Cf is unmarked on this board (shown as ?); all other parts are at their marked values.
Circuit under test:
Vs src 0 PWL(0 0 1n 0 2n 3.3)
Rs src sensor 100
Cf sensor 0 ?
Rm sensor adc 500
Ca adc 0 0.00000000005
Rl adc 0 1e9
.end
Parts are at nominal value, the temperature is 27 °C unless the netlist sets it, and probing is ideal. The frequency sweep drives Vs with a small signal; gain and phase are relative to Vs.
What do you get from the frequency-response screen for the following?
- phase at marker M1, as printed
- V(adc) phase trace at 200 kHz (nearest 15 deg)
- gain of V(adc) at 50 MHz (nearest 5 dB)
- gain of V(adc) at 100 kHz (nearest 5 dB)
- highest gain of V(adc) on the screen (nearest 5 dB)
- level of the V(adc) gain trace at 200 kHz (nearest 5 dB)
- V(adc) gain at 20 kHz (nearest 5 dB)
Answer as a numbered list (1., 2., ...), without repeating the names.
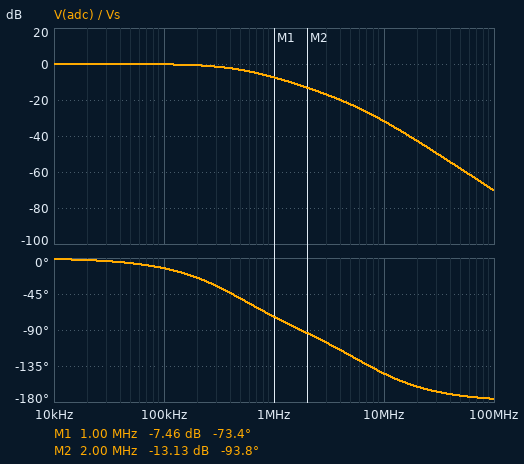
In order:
1. -73.4 deg
2. -30 deg
3. -60 dB
4. 0 dB
5. 0 dB
6. 0 dB
7. 0 dB
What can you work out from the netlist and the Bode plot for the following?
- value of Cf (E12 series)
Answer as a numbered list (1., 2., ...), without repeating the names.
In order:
1. 3.3 nF
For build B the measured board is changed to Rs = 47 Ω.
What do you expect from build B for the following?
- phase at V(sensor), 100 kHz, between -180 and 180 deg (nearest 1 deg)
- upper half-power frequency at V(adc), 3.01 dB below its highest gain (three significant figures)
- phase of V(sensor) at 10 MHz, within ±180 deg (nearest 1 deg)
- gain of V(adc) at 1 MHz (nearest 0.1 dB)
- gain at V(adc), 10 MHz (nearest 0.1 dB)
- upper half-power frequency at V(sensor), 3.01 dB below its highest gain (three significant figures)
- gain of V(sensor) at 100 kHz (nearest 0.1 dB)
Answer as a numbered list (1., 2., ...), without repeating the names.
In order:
1. -6 deg
2. 985 kHz
3. -84 deg
4. -3.1 dB
5. -25.3 dB
6. 1.01 MHz
7. 0 dB
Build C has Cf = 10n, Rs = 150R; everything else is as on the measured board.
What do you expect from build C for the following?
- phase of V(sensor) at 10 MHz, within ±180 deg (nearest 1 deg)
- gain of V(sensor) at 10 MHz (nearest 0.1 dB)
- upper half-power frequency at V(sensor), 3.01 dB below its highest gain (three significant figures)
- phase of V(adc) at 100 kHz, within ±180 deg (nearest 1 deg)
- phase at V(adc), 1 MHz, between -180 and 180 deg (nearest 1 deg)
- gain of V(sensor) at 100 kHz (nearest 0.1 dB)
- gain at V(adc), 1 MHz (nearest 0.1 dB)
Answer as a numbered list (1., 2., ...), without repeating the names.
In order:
1. -89 deg
2. -39.5 dB
3. 106 kHz
4. -44 deg
5. -93 deg
6. -2.8 dB
7. -19.7 dB
